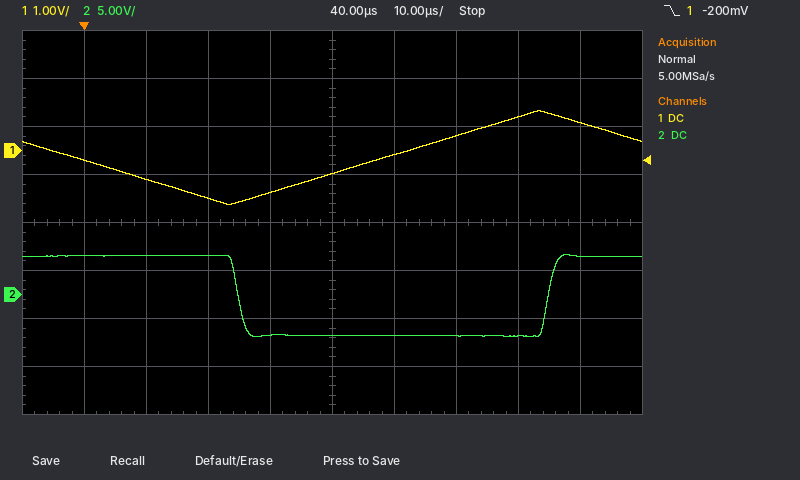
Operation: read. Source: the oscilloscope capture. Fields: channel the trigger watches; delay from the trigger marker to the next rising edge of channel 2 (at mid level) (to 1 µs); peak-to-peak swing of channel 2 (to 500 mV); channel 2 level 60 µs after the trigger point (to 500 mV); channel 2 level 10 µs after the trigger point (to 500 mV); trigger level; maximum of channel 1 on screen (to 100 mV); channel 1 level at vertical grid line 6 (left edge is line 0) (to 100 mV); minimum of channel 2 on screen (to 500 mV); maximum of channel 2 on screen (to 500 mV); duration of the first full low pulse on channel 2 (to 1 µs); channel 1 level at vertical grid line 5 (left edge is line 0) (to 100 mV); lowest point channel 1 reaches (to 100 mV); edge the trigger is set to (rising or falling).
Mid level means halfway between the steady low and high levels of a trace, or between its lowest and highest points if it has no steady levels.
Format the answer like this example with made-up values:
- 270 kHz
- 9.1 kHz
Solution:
- channel 1
- 75 µs
- 8.5 V
- -4.5 V
- 4.0 V
- -200 mV
- 800 mV
- -100 mV
- -4.5 V
- 4.0 V
- 50 µs
- -500 mV
- -1.1 V
- falling
